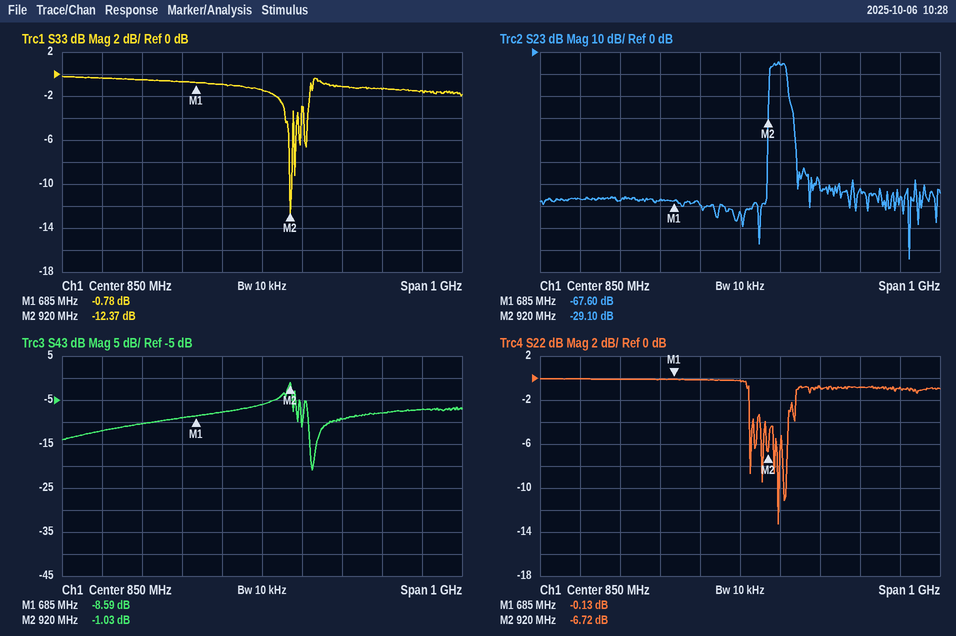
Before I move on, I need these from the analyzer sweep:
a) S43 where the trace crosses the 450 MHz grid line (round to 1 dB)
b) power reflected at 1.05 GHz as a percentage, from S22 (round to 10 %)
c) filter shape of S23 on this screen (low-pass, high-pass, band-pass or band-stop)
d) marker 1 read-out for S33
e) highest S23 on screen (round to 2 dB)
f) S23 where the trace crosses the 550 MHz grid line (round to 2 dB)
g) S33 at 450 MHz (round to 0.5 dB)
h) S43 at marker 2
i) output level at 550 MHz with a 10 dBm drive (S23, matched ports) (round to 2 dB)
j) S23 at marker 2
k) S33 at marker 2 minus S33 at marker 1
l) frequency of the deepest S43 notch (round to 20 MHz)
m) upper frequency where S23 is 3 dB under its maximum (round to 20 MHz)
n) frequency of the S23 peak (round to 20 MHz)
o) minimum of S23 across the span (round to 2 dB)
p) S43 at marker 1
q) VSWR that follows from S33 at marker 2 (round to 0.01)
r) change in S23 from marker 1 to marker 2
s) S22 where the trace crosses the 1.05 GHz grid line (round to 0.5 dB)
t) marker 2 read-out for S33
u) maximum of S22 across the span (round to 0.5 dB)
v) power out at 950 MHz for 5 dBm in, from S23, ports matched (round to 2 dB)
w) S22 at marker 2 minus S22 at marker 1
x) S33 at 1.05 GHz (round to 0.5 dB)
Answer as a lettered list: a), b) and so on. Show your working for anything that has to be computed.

a) -12 dB
b) 10^(-1/10) ≈ 79.4 %, so 80 % to the nearest 10 %
c) band-pass
d) -0.78 dB
e) -4 dB
f) -68 dB
g) -0.5 dB
h) -1.03 dB
i) 10 dBm + (-68 dB) = -58 dBm
j) -29.10 dB
k) -12.37 − (-0.78) = -11.59 dB
l) 980 MHz
m) 960 MHz
n) 940 MHz
o) -94 dB
p) -8.59 dB
q) (1 + 0.2407)/(1 − 0.2407) ≈ 1.63
r) -29.1 − (-67.6) = 38.50 dB
s) -1.0 dB
t) -12.37 dB
u) 0.0 dB
v) 5 dBm + (-6 dB) = 0 dBm
w) -6.72 − (-0.13) = -6.59 dB
x) -1.0 dB
